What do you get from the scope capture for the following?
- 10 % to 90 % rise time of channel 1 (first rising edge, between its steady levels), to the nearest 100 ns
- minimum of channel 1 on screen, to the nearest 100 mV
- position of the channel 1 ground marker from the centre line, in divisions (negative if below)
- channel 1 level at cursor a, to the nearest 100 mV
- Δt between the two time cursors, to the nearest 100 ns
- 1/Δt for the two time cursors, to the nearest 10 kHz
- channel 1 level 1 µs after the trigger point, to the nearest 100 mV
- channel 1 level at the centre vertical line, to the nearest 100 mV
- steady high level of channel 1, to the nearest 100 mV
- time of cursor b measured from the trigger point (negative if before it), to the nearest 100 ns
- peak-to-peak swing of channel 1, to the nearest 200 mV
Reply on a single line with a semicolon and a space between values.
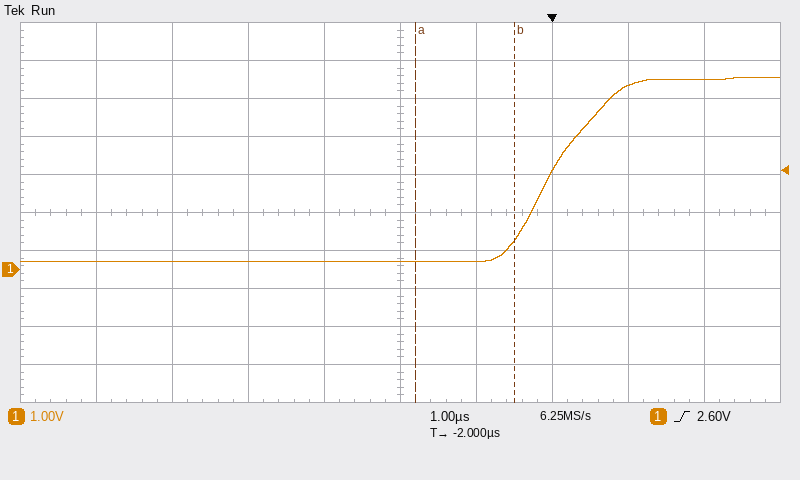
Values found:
1.3 µs; 200 mV; -1.5 div; 200 mV; 1.3 µs; 770 kHz; 4.8 V; 200 mV; 5.0 V; -500 ns; 4.8 V
